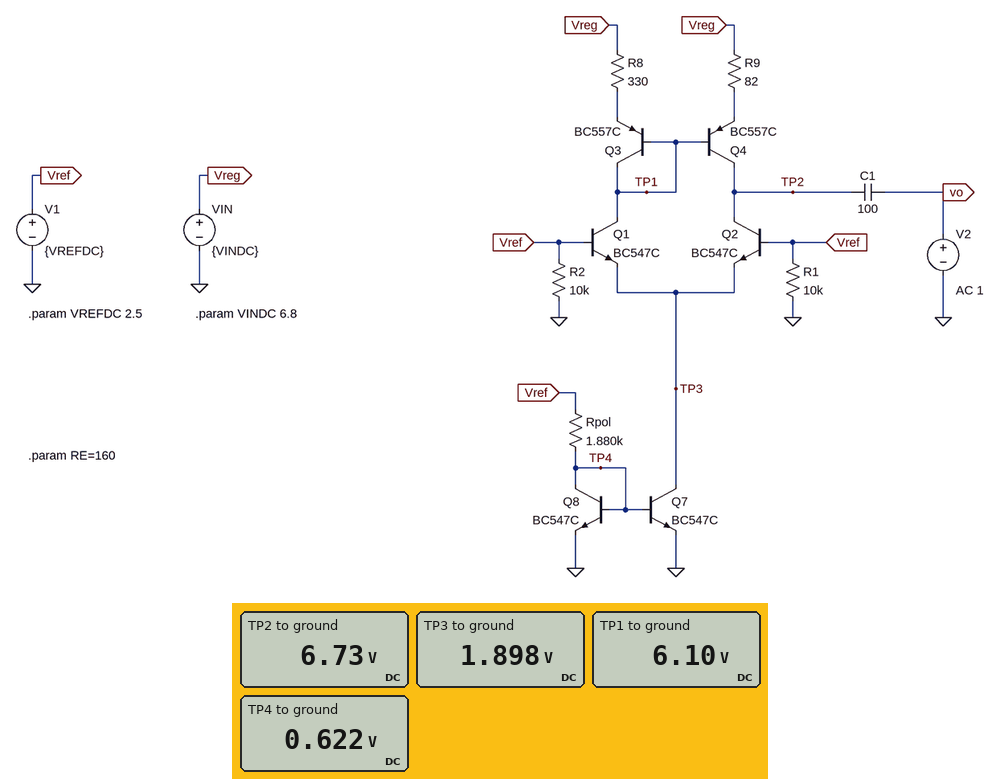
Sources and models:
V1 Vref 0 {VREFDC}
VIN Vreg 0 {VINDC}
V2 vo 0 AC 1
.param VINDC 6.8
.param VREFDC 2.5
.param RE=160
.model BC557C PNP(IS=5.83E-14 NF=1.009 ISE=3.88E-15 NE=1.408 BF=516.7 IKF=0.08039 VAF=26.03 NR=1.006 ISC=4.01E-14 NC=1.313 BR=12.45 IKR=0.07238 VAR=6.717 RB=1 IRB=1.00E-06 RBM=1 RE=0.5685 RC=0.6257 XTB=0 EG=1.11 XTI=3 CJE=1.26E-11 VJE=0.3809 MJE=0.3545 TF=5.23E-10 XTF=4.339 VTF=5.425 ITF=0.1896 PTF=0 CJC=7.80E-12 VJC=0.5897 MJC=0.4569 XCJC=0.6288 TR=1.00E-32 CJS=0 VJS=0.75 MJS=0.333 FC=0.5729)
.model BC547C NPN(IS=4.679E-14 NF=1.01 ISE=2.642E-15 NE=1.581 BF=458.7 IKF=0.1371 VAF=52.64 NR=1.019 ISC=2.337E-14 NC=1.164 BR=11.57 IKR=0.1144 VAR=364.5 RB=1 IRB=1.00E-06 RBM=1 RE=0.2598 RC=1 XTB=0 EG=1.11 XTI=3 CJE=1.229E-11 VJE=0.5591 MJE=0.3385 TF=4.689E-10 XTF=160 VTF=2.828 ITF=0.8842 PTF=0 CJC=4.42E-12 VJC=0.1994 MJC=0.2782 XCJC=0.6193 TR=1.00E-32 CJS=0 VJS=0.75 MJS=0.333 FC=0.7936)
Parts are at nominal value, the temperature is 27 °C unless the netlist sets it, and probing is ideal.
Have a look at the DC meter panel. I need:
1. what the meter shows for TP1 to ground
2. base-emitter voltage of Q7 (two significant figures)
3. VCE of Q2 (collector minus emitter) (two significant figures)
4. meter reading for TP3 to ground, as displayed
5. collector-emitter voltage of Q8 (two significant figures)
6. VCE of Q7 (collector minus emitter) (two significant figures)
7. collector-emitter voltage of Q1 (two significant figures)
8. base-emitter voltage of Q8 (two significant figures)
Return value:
6.10 V
620 mV
4.8 V
1.898 V
620 mV
1.9 V
4.2 V
620 mV
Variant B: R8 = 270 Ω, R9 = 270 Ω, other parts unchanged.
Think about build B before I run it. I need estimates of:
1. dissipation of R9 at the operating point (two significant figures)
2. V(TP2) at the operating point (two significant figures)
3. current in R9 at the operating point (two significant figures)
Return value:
70 µW
5.9 V
510 µA
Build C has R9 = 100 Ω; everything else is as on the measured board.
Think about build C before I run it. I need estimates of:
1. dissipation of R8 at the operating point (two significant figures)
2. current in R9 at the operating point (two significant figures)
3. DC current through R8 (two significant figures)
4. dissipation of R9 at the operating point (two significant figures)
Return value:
41 µW
660 µA
350 µA
44 µW
